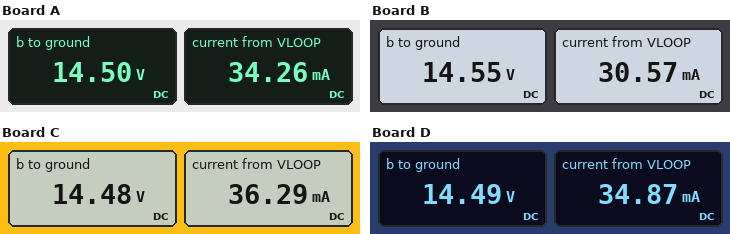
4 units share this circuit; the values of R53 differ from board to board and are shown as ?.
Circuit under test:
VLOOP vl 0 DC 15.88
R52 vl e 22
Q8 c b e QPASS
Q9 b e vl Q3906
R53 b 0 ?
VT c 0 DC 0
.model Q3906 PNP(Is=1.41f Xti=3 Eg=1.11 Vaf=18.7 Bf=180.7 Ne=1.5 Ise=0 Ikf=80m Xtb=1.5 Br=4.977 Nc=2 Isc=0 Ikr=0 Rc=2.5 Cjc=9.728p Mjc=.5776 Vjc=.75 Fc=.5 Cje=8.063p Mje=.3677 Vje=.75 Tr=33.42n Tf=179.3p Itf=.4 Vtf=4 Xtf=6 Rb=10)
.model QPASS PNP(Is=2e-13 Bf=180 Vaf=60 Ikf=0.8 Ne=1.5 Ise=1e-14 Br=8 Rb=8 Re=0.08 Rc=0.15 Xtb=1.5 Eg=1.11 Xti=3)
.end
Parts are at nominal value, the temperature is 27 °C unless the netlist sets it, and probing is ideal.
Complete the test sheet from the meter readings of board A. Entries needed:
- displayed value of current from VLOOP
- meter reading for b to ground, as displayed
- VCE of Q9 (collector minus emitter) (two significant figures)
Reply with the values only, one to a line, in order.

34.26 mA
14.50 V
-1.4 V
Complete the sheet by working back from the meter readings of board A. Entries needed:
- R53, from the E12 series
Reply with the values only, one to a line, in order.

8.2 kΩ
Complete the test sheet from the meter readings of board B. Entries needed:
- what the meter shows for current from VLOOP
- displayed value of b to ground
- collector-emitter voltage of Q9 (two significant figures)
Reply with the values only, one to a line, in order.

30.57 mA
14.55 V
-1.3 V
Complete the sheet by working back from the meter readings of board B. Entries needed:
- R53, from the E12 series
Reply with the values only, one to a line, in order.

39 kΩ
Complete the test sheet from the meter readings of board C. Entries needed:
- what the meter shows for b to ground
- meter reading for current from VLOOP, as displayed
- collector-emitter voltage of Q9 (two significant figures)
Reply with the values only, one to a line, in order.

14.48 V
36.29 mA
-1.4 V
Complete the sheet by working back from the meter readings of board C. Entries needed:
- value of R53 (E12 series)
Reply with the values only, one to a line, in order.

4.7 kΩ
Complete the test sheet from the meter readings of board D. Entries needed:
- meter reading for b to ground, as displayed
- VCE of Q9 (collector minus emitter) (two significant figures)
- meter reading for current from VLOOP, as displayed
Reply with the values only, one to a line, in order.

14.49 V
-1.4 V
34.87 mA
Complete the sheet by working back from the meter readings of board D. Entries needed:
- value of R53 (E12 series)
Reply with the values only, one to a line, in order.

6.8 kΩ
